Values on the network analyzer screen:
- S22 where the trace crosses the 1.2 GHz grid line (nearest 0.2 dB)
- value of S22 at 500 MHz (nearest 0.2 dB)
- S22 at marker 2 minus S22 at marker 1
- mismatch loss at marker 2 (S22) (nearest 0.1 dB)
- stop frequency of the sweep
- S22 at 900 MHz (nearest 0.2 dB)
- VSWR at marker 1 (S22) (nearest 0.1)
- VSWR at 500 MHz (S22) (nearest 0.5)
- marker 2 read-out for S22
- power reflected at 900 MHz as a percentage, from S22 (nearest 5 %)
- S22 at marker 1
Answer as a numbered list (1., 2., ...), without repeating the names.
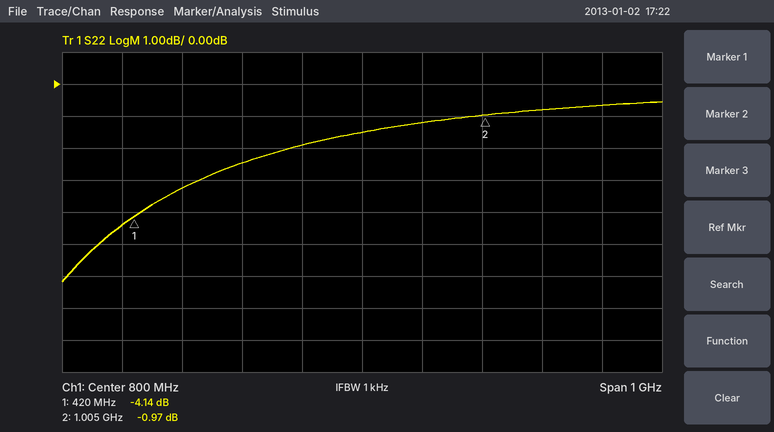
1. -0.6 dB
2. -3.2 dB
3. 3.17 dB
4. 7.0 dB
5. 1.3 GHz
6. -1.2 dB
7. 4.3
8. 5.5
9. -0.97 dB
10. 75 %
11. -4.14 dB
